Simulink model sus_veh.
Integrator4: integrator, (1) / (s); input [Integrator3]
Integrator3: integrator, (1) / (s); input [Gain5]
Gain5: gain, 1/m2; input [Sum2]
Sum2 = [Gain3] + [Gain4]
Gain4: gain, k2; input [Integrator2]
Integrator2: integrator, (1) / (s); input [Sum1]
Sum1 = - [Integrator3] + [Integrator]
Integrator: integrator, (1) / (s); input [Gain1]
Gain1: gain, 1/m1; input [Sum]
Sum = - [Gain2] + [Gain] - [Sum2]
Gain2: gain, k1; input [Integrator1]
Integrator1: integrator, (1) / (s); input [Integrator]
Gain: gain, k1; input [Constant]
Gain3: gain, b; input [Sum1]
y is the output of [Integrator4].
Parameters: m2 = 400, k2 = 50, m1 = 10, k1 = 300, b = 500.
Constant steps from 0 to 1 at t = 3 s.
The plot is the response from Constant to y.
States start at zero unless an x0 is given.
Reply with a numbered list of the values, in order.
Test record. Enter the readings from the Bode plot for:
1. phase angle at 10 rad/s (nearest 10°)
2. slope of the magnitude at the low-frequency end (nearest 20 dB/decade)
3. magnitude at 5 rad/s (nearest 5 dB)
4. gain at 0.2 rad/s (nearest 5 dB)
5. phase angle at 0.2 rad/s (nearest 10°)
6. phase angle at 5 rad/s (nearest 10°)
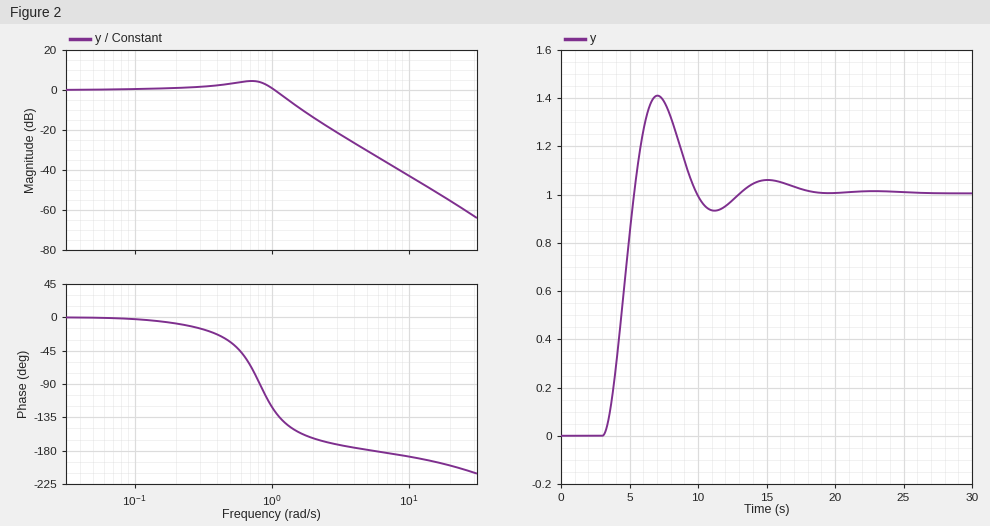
1. -190°
2. 0 dB/decade
3. -30 dB
4. 0 dB
5. -10°
6. -180°
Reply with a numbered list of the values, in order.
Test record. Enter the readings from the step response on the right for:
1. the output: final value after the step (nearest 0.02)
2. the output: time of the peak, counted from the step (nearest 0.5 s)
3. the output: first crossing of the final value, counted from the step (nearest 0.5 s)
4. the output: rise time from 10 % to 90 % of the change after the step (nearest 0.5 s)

1. 1.00
2. 4.0 s
3. 2.5 s
4. 1.5 s
